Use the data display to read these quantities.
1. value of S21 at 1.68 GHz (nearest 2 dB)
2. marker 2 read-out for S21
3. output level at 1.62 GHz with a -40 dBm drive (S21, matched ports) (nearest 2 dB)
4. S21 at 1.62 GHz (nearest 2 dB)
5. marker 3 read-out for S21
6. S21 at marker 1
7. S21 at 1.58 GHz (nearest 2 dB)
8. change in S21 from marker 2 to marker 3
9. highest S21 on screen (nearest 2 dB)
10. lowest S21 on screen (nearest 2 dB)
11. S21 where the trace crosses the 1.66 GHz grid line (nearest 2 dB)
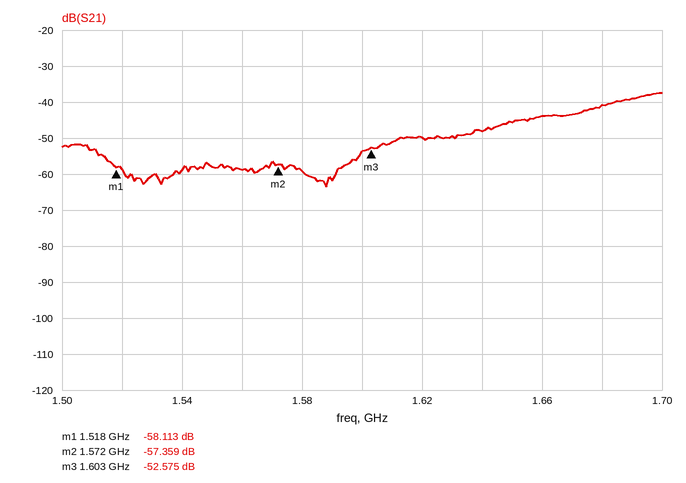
-40 dB
-57.359 dB
-90 dBm
-50 dB
-52.575 dB
-58.113 dB
-60 dB
4.784 dB
-38 dB
-64 dB
-44 dB
